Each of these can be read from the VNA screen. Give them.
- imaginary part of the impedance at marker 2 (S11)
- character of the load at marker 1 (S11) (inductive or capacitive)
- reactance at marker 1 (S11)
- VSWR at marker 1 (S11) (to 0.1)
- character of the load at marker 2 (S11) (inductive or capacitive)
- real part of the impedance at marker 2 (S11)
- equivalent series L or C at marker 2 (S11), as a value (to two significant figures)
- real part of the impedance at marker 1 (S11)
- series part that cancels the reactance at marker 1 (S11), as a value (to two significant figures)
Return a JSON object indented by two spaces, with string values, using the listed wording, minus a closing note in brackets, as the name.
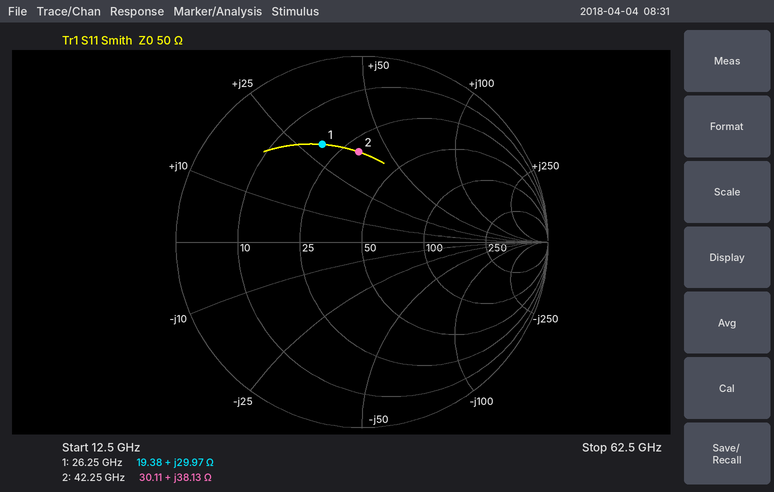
{
  "imaginary part of the impedance at marker 2": "+38.13 Ω",
  "character of the load at marker 1 (S11)": "inductive",
  "reactance at marker 1": "+29.97 Ω",
  "VSWR at marker 1 (S11)": "3.6",
  "character of the load at marker 2 (S11)": "inductive",
  "real part of the impedance at marker 2": "30.11 Ω",
  "equivalent series L or C at marker 2 (S11), as a value": "140 pH",
  "real part of the impedance at marker 1": "19.38 Ω",
  "series part that cancels the reactance at marker 1 (S11), as a value": "200 fF"
}
